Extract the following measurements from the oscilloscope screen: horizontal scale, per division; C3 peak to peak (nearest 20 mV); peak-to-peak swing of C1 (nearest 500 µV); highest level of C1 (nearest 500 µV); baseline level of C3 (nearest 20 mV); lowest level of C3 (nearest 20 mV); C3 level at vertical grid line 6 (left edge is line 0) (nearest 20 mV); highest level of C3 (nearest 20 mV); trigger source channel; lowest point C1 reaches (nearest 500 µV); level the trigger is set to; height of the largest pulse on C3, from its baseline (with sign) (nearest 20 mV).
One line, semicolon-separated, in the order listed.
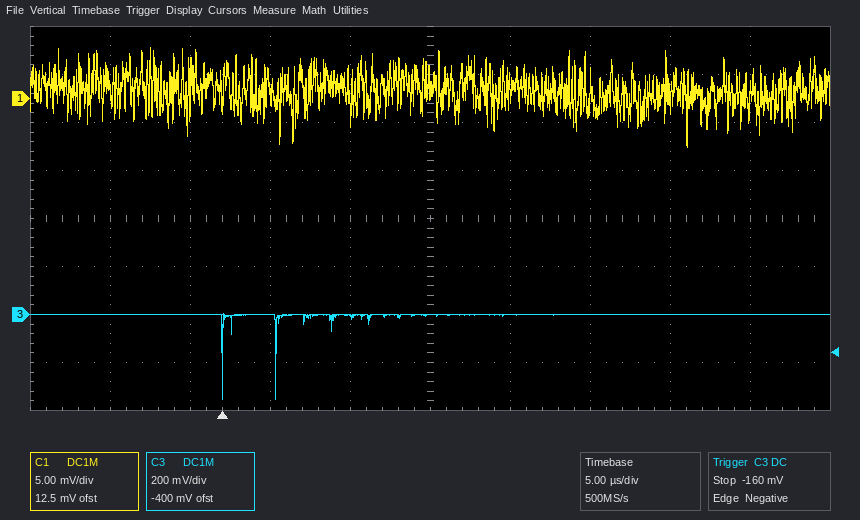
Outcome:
5 µs; 360 mV; 10.5 mV; 5.5 mV; 0 mV; -360 mV; 0 mV; 0 mV; C3; -5.0 mV; -160 mV; -360 mV
